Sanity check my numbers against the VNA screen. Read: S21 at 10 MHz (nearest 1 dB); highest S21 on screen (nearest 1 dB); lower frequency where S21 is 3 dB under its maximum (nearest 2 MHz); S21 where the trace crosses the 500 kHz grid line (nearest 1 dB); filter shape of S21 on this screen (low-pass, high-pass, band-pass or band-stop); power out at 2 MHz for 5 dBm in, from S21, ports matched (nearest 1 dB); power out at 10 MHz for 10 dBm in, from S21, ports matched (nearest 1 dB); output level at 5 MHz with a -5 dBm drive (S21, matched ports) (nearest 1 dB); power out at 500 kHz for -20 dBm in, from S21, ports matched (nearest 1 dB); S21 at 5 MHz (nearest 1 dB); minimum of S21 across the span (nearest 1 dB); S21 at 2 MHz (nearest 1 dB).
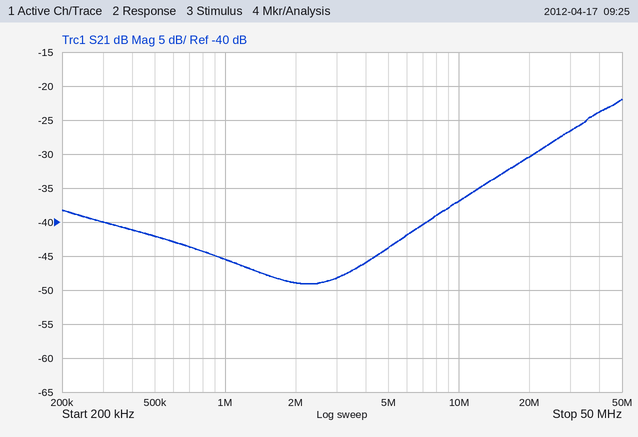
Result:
-37 dB
-22 dB
36 MHz
-42 dB
high-pass
-44 dBm
-27 dBm
-49 dBm
-62 dBm
-44 dB
-49 dB
-49 dB
